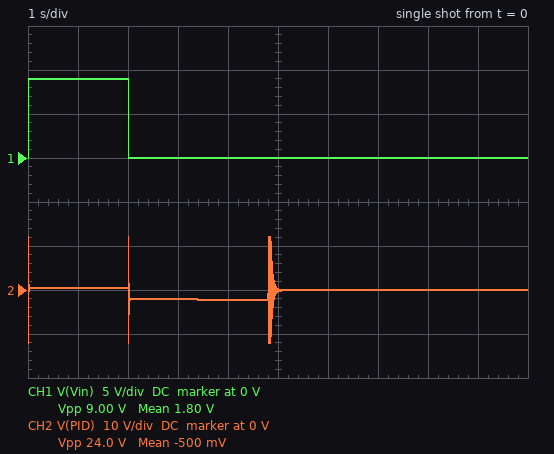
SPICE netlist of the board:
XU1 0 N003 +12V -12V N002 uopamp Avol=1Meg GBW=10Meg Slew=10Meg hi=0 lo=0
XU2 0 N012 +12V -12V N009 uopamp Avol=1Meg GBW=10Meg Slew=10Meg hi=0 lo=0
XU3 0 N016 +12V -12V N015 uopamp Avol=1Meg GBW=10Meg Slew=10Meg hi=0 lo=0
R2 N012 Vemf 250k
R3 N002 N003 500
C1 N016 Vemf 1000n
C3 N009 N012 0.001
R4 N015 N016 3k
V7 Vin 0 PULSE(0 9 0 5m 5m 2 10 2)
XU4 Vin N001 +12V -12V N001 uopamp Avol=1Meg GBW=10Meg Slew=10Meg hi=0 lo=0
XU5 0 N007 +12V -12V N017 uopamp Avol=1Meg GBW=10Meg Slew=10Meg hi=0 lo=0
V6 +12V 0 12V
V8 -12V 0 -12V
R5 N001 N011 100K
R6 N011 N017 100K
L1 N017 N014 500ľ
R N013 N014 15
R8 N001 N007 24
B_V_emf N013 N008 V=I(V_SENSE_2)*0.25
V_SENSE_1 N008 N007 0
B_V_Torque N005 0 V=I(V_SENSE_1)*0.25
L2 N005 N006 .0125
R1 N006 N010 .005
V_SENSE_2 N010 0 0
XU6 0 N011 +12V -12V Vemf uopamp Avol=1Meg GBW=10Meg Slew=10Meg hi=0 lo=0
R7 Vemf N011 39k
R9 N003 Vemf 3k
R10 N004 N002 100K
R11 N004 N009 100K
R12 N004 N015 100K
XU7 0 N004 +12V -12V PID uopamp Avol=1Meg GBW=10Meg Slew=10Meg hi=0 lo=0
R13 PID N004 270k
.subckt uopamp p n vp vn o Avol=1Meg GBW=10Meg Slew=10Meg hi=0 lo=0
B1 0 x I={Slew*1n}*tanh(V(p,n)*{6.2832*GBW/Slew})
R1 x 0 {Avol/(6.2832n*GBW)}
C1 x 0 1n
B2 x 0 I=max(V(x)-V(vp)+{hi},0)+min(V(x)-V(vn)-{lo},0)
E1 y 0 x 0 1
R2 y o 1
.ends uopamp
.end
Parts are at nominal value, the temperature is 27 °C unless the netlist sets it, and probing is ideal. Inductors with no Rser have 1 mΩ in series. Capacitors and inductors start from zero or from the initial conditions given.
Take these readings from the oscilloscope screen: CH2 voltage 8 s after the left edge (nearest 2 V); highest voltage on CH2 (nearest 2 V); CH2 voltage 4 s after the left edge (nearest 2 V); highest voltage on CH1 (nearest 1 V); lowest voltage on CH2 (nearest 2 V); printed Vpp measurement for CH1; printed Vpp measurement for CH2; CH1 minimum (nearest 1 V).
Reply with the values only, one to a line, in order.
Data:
0 V
12 V
-2 V
9 V
-12 V
9.00 V
24.0 V
0 V
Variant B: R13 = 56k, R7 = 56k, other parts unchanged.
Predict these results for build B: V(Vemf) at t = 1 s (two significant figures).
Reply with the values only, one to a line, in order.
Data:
1.7 V
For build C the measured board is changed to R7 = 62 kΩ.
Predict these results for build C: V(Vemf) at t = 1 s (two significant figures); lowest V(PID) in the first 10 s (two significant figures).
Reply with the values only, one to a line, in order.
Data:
1.8 V
-12 V
